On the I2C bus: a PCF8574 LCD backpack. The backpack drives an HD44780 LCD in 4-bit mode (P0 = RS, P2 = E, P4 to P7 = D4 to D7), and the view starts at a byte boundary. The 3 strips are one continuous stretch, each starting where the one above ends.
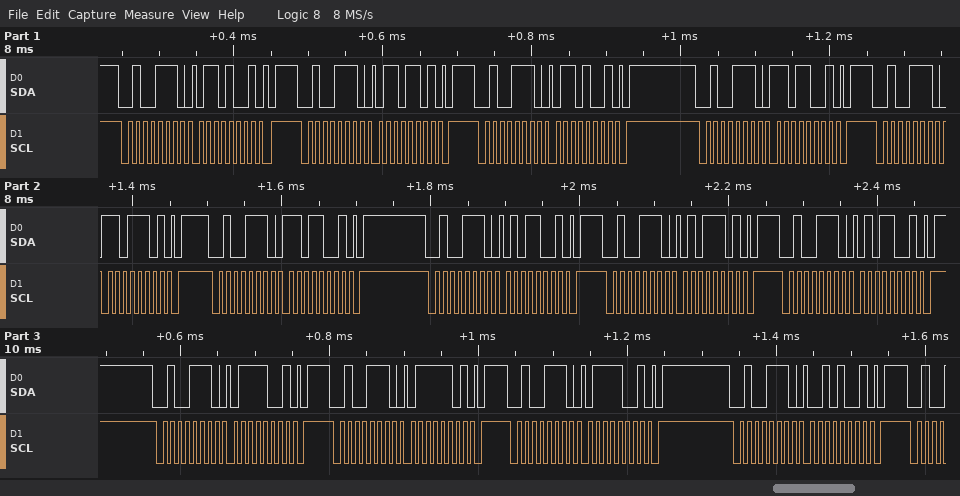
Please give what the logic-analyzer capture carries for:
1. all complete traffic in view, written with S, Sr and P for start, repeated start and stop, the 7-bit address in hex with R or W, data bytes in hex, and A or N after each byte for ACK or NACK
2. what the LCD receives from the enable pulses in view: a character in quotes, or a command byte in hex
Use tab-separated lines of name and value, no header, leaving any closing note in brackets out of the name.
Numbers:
all complete traffic in view, written with S, Sr and P for start, repeated start and stop, the 7-bit address in hex with R or W, data bytes in hex, and A or N after each byte for ACK or NACK	S 27W A 69 A P S 27W A 6D A P S 27W A 69 A P S 27W A D9 A P S 27W A DD A P S 27W A D9 A P S 27W A 59 A P S 27W A 5D A P S 27W A 59 A P S 27W A 79 A P S 27W A 7D A P S 27W A 79 A P S 27W A 29 A P
what the LCD receives from the enable pulses in view: a character in quotes, or a command byte in hex	'm' 'W'
